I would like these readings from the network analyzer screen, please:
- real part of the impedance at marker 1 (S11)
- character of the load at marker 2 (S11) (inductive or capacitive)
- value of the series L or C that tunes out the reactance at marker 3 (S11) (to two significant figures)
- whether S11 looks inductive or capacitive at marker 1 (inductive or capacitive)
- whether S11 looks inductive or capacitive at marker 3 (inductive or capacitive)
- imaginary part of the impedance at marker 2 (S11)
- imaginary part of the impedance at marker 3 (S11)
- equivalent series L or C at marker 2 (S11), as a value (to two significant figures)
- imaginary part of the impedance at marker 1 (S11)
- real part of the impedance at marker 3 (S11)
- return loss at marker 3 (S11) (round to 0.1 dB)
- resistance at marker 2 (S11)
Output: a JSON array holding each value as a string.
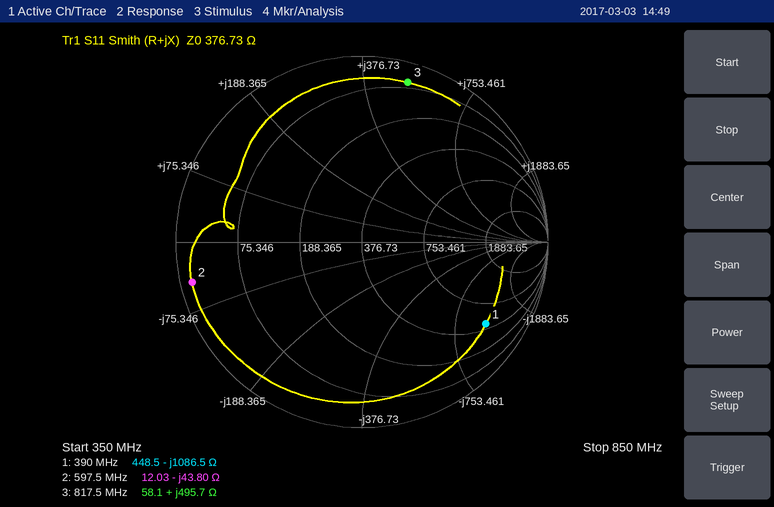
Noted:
["448.5 Ω", "capacitive", "390 fF", "capacitive", "inductive", "-43.80 Ω", "+495.7 Ω", "6.1 pF", "-1086.5 Ω", "58.1 Ω", "1.0 dB", "12.03 Ω"]
